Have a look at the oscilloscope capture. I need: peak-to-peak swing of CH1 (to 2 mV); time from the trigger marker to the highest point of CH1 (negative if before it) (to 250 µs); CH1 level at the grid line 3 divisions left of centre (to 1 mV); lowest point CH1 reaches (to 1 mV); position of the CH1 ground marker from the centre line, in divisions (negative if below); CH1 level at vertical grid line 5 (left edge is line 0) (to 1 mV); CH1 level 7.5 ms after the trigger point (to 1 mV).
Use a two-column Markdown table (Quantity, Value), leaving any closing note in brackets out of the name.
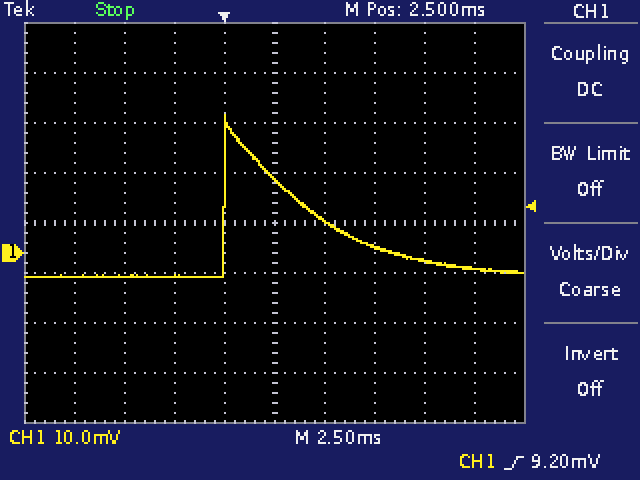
| Quantity | Value |
|---|---|
| peak-to-peak swing of CH1 | 32 mV |
| time from the trigger marker to the highest point of CH1 (negative if before it) | 0.00 ms |
| CH1 level at the grid line 3 divisions left of centre | -5 mV |
| lowest point CH1 reaches | -5 mV |
| position of the CH1 ground marker from the centre line, in divisions | -0.6 div |
| CH1 level at vertical grid line 5 (left edge is line 0) | 15 mV |
| CH1 level 7.5 ms after the trigger point | 1 mV |
